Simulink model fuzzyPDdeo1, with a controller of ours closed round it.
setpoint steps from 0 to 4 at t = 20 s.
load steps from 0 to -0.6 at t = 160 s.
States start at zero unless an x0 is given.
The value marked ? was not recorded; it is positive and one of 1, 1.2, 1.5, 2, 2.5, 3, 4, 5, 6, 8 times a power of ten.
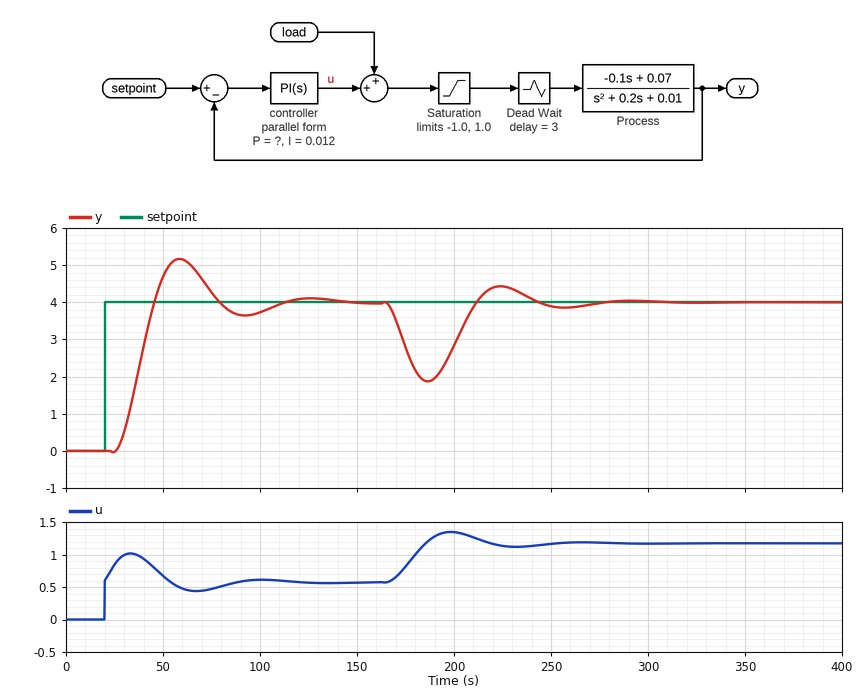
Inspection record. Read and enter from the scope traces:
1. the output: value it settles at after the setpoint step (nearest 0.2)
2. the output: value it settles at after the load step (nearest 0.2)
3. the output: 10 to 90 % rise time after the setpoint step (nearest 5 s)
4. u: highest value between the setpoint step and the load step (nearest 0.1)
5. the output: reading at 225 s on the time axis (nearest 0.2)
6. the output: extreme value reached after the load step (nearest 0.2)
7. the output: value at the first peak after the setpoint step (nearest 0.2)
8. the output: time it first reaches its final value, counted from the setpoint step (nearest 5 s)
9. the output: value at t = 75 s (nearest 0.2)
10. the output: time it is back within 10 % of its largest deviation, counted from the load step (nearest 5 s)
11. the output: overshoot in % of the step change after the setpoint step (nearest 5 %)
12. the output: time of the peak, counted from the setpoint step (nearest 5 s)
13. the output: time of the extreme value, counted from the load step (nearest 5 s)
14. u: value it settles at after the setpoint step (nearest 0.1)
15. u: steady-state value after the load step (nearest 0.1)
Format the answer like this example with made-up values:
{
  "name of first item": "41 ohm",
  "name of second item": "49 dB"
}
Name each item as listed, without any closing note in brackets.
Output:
{
  "the output: value it settles at after the setpoint step": "4.0",
  "the output: value it settles at after the load step": "4.0",
  "the output: 10 to 90 % rise time after the setpoint step": "15 s",
  "u: highest value between the setpoint step and the load step": "1.0",
  "the output: reading at 225 s on the time axis": "4.4",
  "the output: extreme value reached after the load step": "1.8",
  "the output: value at the first peak after the setpoint step": "5.2",
  "the output: time it first reaches its final value, counted from the setpoint step": "25 s",
  "the output: value at t = 75 s": "4.2",
  "the output: time it is back within 10 % of its largest deviation, counted from the load step": "75 s",
  "the output: overshoot in % of the step change after the setpoint step": "30 %",
  "the output: time of the peak, counted from the setpoint step": "40 s",
  "the output: time of the extreme value, counted from the load step": "25 s",
  "u: value it settles at after the setpoint step": "0.6",
  "u: steady-state value after the load step": "1.2"
}
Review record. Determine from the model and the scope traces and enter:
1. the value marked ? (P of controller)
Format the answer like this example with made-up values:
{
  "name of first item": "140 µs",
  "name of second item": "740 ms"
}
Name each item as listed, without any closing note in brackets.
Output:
{
  "the value marked ?": "0.15"
}
